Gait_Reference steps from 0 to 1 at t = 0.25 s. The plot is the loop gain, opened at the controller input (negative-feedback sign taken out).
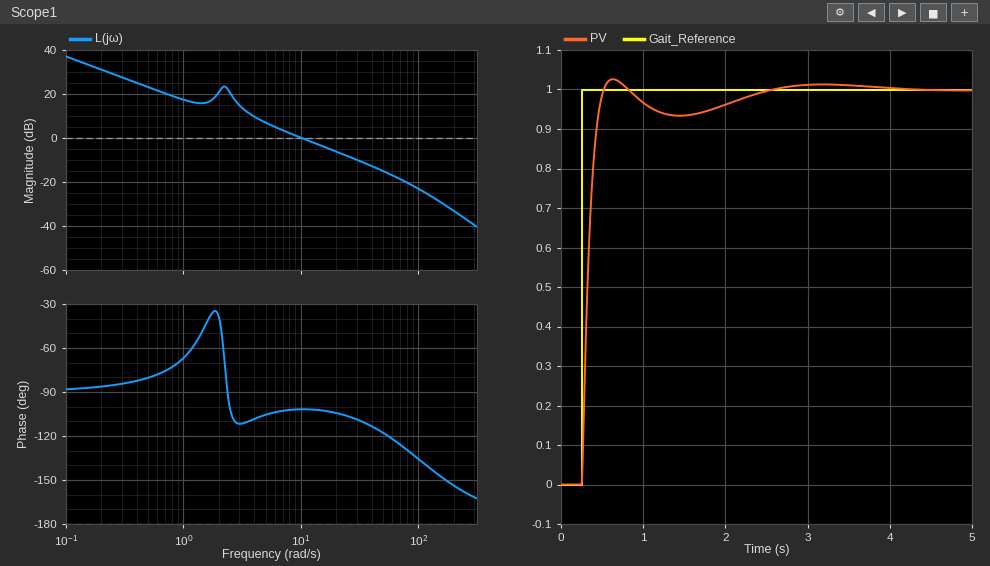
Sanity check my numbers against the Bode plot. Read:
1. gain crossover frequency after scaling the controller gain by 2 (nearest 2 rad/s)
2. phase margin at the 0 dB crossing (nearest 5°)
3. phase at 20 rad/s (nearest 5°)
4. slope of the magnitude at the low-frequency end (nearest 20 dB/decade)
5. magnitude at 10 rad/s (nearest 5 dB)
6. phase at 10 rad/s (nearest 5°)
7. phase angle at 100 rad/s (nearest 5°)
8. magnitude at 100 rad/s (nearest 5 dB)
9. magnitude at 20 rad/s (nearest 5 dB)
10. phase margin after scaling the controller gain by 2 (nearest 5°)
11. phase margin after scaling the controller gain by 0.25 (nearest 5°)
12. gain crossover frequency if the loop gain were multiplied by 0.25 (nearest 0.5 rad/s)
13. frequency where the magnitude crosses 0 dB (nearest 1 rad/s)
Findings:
20 rad/s
80°
-105°
-20 dB/decade
0 dB
-100°
-135°
-25 dB
-5 dB
75°
70°
3.5 rad/s
10 rad/s
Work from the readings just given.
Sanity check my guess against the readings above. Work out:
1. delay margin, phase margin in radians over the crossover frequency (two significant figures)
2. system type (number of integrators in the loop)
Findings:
0.14 s
1
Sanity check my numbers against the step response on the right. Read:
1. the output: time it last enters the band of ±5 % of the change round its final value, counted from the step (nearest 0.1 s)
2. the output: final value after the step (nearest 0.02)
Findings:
1.6 s
1.00
